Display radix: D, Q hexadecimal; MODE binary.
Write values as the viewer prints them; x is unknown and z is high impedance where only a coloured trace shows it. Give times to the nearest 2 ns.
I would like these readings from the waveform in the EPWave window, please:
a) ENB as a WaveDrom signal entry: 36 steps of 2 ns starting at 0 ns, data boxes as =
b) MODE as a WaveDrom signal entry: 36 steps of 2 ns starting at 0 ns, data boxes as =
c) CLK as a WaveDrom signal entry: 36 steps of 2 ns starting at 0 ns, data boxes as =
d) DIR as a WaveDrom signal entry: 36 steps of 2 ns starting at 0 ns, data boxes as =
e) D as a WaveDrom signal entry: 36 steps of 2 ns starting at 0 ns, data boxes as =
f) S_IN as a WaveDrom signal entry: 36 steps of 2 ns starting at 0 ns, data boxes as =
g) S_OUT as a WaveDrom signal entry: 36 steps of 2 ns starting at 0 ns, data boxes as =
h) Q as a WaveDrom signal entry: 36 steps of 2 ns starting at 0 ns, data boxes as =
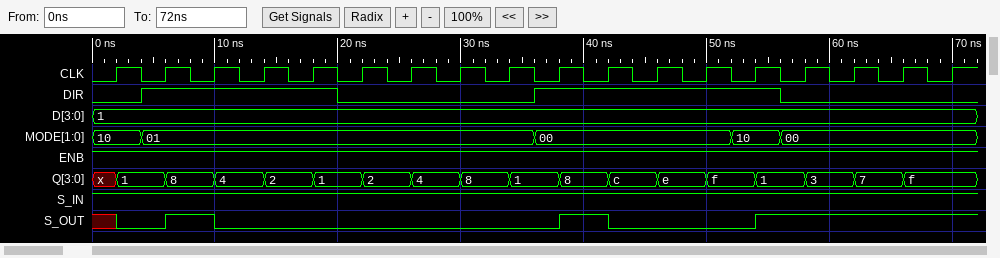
{name: 'ENB', wave: '1...................................'}
{name: 'MODE', wave: '=.=...............=.......=.=.......', data: '10 01 00 10 00'}
{name: 'CLK', wave: '010101010101010101010101010101010101'}
{name: 'DIR', wave: '0.1.......0.......1.........0.......'}
{name: 'D', wave: '=...................................', data: '1'}
{name: 'S_IN', wave: '1...................................'}
{name: 'S_OUT', wave: 'x0.1.0.............1.0.....1........'}
{name: 'Q', wave: 'x=.=.=.=.=.=.=.=.=.=.=.=.=.=.=.=.=..', data: '1 8 4 2 1 2 4 8 1 8 c e f 1 3 7 f'}
